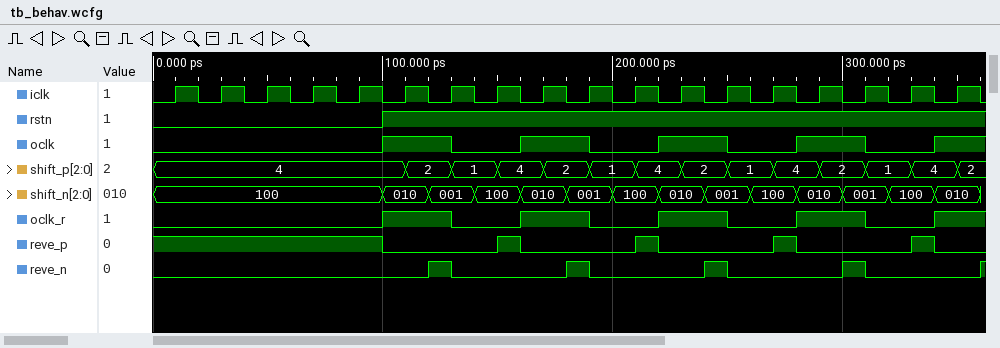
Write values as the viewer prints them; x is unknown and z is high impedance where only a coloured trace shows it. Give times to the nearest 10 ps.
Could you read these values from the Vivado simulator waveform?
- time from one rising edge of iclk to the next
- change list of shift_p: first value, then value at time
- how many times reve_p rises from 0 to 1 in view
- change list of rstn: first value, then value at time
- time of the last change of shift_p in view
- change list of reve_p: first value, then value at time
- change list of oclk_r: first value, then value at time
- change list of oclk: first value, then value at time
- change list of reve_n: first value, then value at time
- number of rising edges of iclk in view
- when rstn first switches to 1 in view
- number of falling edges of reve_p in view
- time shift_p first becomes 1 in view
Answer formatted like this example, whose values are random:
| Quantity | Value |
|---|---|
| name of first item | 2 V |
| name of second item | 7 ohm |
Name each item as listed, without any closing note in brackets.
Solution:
| Quantity | Value |
|---|---|
| time from one rising edge of iclk to the next | 20 ps |
| change list of shift_p: first value, then value at time | 4, 2 at 110 ps, 1 at 130 ps, 4 at 150 ps, 2 at 170 ps, 1 at 190 ps, 4 at 210 ps, 2 at 230 ps, 1 at 250 ps, 4 at 270 ps, 2 at 290 ps, 1 at 310 ps, 4 at 330 ps, 2 at 350 ps |
| how many times reve_p rises from 0 to 1 in view | 4 |
| change list of rstn: first value, then value at time | 0, 1 at 100 ps |
| time of the last change of shift_p in view | 350 ps |
| change list of reve_p: first value, then value at time | 1, 0 at 100 ps, 1 at 150 ps, 0 at 160 ps, 1 at 210 ps, 0 at 220 ps, 1 at 270 ps, 0 at 280 ps, 1 at 330 ps, 0 at 340 ps |
| change list of oclk_r: first value, then value at time | 0, 1 at 100 ps, 0 at 130 ps, 1 at 160 ps, 0 at 190 ps, 1 at 220 ps, 0 at 250 ps, 1 at 280 ps, 0 at 310 ps, 1 at 340 ps |
| change list of oclk: first value, then value at time | 0, 1 at 100 ps, 0 at 130 ps, 1 at 160 ps, 0 at 190 ps, 1 at 220 ps, 0 at 250 ps, 1 at 280 ps, 0 at 310 ps, 1 at 340 ps |
| change list of reve_n: first value, then value at time | 0, 1 at 120 ps, 0 at 130 ps, 1 at 180 ps, 0 at 190 ps, 1 at 240 ps, 0 at 250 ps, 1 at 300 ps, 0 at 310 ps, 1 at 360 ps |
| number of rising edges of iclk in view | 18 |
| when rstn first switches to 1 in view | 100 ps |
| number of falling edges of reve_p in view | 5 |
| time shift_p first becomes 1 in view | 130 ps |
